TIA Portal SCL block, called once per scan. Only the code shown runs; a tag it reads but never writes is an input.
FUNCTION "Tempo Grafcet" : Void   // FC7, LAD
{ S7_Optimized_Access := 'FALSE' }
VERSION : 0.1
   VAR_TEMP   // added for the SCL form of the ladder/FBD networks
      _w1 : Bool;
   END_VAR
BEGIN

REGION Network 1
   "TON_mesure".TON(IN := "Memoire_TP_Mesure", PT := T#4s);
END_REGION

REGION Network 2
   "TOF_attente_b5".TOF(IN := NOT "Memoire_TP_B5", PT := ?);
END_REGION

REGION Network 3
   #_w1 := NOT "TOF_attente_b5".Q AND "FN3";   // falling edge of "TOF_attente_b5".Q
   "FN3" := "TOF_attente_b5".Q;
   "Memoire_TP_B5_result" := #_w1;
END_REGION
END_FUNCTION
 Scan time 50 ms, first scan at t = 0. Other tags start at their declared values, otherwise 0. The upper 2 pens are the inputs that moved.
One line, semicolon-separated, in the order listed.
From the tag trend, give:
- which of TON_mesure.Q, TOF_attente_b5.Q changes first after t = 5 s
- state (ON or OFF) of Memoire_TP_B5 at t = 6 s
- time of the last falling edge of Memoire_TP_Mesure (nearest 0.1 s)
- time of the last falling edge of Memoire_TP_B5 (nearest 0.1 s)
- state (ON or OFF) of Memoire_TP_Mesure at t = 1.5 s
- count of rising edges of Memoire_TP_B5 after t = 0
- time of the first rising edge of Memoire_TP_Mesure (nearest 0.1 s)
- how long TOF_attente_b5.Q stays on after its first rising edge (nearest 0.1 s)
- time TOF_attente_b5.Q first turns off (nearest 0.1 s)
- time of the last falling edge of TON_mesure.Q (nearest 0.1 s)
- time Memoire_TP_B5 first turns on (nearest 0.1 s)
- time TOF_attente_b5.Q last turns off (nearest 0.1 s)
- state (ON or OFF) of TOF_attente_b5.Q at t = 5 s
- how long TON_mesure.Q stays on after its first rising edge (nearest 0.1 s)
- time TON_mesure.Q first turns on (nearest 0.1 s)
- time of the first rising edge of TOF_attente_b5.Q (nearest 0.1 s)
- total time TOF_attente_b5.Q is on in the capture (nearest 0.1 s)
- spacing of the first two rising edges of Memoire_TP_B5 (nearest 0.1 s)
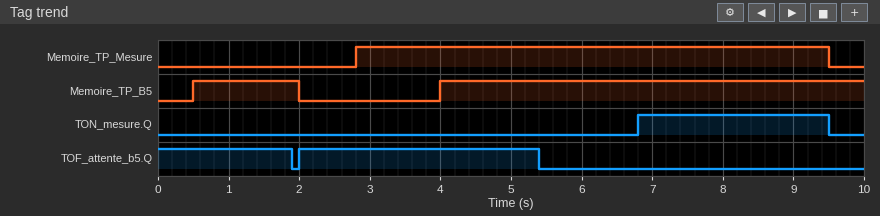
TOF_attente_b5.Q; ON; 9.5 s; 2.0 s; OFF; 2; 2.8 s; 3.4 s; 1.9 s; 9.5 s; 0.5 s; 5.4 s; ON; 2.7 s; 6.8 s; 2.0 s; 5.3 s; 3.5 s
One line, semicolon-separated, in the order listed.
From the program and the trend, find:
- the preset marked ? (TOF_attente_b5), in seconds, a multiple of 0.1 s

1.4 s
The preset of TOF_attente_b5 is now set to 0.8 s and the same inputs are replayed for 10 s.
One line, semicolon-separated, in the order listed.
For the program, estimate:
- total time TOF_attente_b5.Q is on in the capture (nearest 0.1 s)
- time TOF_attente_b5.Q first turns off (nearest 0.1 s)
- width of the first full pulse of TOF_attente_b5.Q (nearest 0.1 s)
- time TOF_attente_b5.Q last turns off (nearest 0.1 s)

4.1 s; 1.3 s; 2.8 s; 4.8 s
